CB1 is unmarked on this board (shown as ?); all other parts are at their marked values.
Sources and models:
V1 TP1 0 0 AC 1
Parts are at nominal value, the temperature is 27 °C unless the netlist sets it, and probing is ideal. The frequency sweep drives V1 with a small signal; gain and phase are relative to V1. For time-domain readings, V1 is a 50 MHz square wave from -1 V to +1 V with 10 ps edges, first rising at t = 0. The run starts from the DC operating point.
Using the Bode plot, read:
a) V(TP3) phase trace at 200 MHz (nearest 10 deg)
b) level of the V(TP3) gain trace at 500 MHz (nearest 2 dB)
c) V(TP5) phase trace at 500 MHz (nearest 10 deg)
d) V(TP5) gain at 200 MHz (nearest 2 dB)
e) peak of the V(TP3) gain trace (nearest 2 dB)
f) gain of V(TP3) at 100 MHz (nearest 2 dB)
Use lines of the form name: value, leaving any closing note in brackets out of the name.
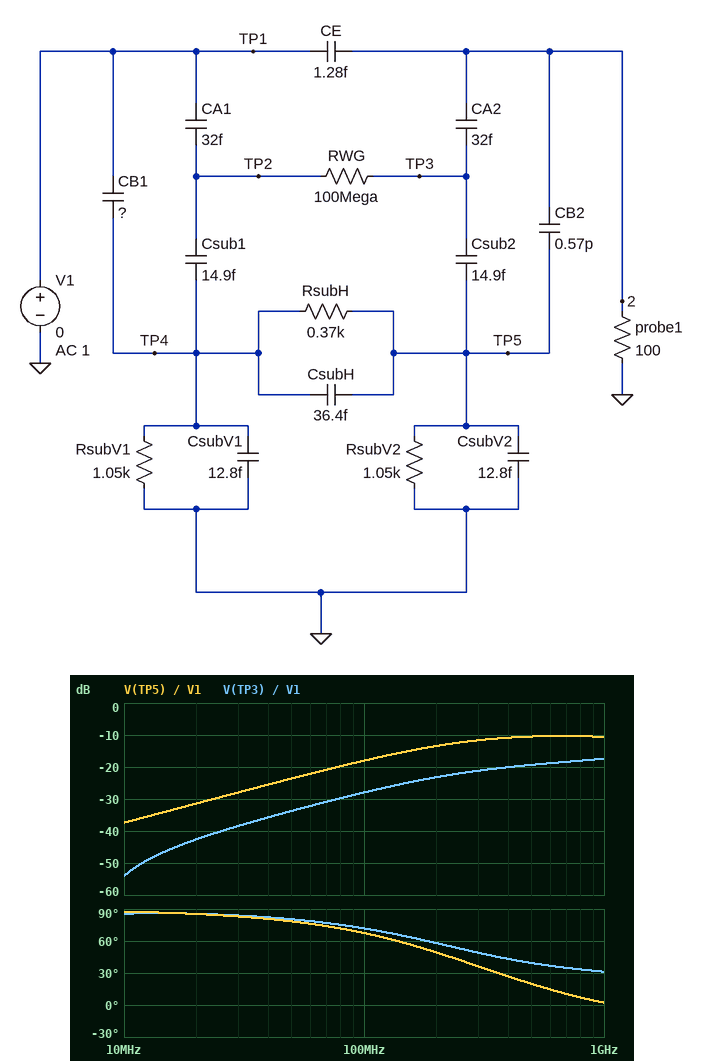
V(TP3) phase trace at 200 MHz: 60 deg
level of the V(TP3) gain trace at 500 MHz: -20 dB
V(TP5) phase trace at 500 MHz: 20 deg
V(TP5) gain at 200 MHz: -14 dB
peak of the V(TP3) gain trace: -18 dB
gain of V(TP3) at 100 MHz: -28 dB
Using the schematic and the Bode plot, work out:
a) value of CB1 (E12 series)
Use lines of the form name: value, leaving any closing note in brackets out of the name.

value of CB1: 470 fF
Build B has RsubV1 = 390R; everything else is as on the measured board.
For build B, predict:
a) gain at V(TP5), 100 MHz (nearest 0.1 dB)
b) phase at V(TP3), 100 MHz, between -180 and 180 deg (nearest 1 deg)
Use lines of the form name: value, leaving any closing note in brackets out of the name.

gain at V(TP5), 100 MHz: -23.6 dB
phase at V(TP3), 100 MHz, between -180 and 180 deg: 80 deg
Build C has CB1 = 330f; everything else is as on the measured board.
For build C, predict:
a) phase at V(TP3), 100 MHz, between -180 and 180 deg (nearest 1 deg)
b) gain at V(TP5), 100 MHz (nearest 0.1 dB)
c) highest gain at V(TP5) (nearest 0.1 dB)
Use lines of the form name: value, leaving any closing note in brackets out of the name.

phase at V(TP3), 100 MHz, between -180 and 180 deg: 75 deg
gain at V(TP5), 100 MHz: -20.9 dB
highest gain at V(TP5): -12.1 dB
